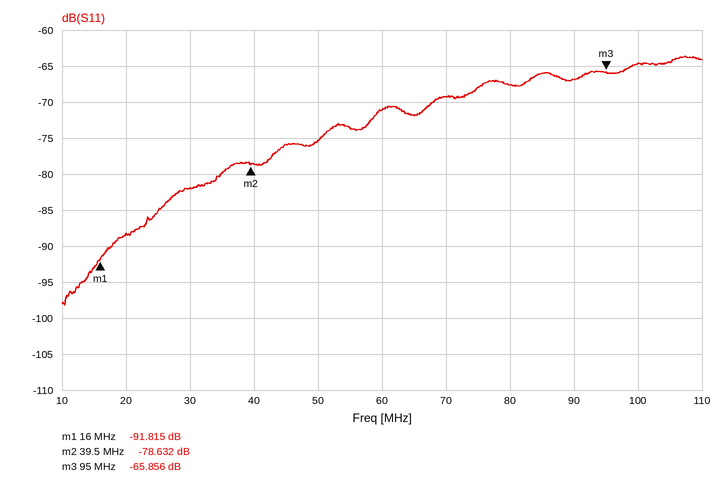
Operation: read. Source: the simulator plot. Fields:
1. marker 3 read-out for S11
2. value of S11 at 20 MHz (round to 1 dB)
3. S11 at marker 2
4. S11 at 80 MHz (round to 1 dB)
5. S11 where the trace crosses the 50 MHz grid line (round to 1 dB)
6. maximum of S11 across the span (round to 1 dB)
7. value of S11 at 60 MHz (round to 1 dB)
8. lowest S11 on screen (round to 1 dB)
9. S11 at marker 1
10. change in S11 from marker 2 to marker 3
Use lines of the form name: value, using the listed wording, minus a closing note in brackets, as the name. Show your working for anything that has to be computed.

marker 3 read-out for S11: -65.856 dB
value of S11 at 20 MHz: -88 dB
S11 at marker 2: -78.632 dB
S11 at 80 MHz: -68 dB
S11 where the trace crosses the 50 MHz grid line: -75 dB
maximum of S11 across the span: -64 dB
value of S11 at 60 MHz: -71 dB
lowest S11 on screen: -98 dB
S11 at marker 1: -91.815 dB
change in S11 from marker 2 to marker 3: -65.856 − (-78.632) = 12.776 dB
